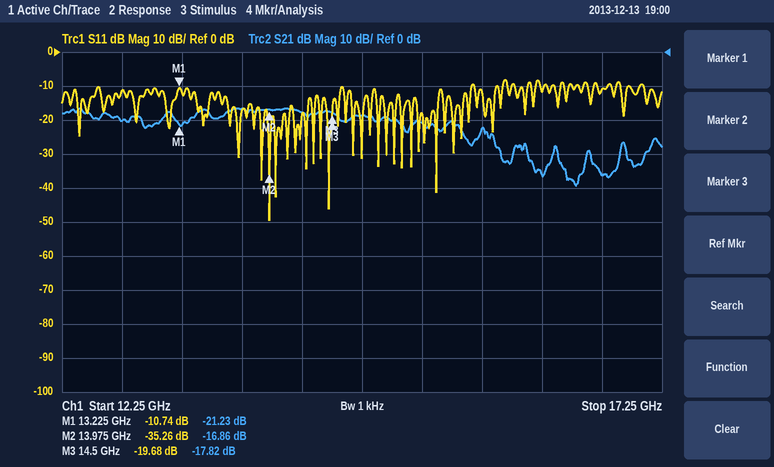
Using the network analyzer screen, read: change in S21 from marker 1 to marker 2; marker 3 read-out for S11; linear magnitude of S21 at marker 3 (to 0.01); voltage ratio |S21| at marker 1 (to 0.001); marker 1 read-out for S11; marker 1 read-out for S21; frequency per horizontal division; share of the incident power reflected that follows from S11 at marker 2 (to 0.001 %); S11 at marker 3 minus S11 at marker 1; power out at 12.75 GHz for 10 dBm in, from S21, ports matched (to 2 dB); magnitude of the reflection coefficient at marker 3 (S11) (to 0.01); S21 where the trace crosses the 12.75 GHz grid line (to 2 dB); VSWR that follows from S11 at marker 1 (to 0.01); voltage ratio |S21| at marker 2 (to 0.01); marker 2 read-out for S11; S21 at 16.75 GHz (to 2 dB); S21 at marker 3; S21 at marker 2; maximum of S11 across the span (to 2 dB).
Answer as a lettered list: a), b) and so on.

a) 4.37 dB
b) -19.68 dB
c) 0.13
d) 0.087
e) -10.74 dB
f) -21.23 dB
g) 500 MHz
h) 0.030 %
i) -8.94 dB
j) -10 dBm
k) 0.10
l) -20 dB
m) 1.82
n) 0.14
o) -35.26 dB
p) -36 dB
q) -17.82 dB
r) -16.86 dB
s) -8 dB
